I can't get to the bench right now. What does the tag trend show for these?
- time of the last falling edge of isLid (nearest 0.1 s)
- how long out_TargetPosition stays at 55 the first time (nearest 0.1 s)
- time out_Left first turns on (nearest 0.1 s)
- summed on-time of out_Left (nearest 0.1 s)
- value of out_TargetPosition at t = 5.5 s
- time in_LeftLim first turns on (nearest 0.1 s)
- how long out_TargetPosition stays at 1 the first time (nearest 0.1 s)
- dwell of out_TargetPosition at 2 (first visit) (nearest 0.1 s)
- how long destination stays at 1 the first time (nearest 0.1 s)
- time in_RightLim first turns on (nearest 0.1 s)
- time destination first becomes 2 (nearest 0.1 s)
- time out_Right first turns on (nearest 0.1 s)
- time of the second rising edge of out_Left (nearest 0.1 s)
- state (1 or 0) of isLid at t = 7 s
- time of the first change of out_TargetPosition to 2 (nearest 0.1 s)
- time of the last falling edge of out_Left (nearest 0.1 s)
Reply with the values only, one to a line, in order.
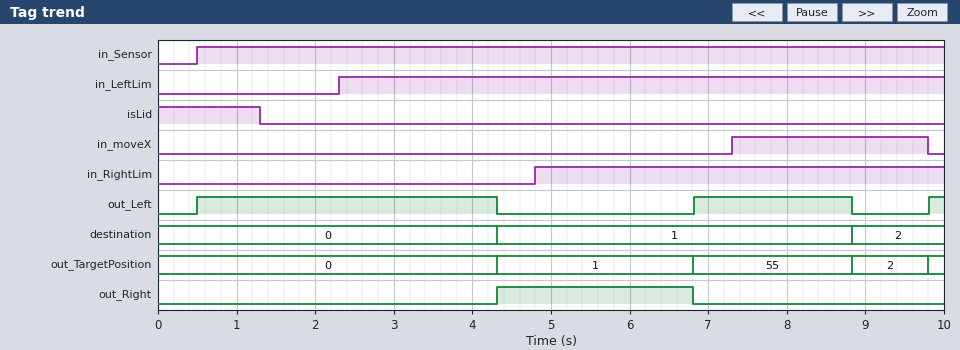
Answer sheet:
1.3 s
2.0 s
0.5 s
6.0 s
1
2.3 s
2.5 s
1.0 s
4.5 s
4.8 s
8.8 s
4.3 s
6.8 s
0
8.8 s
8.8 s
